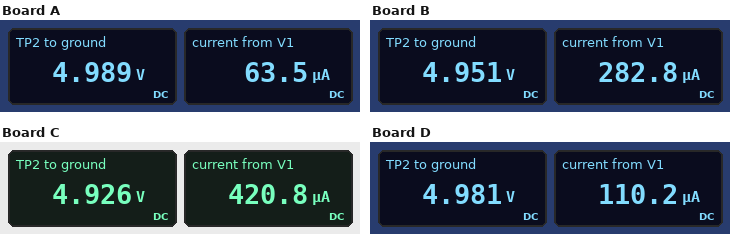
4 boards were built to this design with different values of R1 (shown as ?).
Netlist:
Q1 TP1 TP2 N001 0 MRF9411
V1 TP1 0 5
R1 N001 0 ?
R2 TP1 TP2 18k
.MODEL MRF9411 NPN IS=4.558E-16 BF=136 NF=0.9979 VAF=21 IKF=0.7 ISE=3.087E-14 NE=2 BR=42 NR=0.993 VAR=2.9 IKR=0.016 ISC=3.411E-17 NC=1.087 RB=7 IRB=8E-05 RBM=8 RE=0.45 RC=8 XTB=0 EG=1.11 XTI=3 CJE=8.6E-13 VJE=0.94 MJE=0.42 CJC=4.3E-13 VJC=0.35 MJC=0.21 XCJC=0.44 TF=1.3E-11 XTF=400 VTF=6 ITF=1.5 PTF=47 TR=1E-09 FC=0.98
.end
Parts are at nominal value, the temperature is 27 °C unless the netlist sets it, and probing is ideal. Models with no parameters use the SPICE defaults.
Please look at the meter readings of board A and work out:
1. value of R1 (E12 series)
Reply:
68 kΩ
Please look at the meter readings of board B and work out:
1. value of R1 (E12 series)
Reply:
15 kΩ
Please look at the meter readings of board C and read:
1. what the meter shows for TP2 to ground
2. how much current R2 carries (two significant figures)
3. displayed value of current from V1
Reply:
4.926 V
4.1 µA
420.8 µA
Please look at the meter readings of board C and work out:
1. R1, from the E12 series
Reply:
10 kΩ
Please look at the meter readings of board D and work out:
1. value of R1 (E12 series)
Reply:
39 kΩ
